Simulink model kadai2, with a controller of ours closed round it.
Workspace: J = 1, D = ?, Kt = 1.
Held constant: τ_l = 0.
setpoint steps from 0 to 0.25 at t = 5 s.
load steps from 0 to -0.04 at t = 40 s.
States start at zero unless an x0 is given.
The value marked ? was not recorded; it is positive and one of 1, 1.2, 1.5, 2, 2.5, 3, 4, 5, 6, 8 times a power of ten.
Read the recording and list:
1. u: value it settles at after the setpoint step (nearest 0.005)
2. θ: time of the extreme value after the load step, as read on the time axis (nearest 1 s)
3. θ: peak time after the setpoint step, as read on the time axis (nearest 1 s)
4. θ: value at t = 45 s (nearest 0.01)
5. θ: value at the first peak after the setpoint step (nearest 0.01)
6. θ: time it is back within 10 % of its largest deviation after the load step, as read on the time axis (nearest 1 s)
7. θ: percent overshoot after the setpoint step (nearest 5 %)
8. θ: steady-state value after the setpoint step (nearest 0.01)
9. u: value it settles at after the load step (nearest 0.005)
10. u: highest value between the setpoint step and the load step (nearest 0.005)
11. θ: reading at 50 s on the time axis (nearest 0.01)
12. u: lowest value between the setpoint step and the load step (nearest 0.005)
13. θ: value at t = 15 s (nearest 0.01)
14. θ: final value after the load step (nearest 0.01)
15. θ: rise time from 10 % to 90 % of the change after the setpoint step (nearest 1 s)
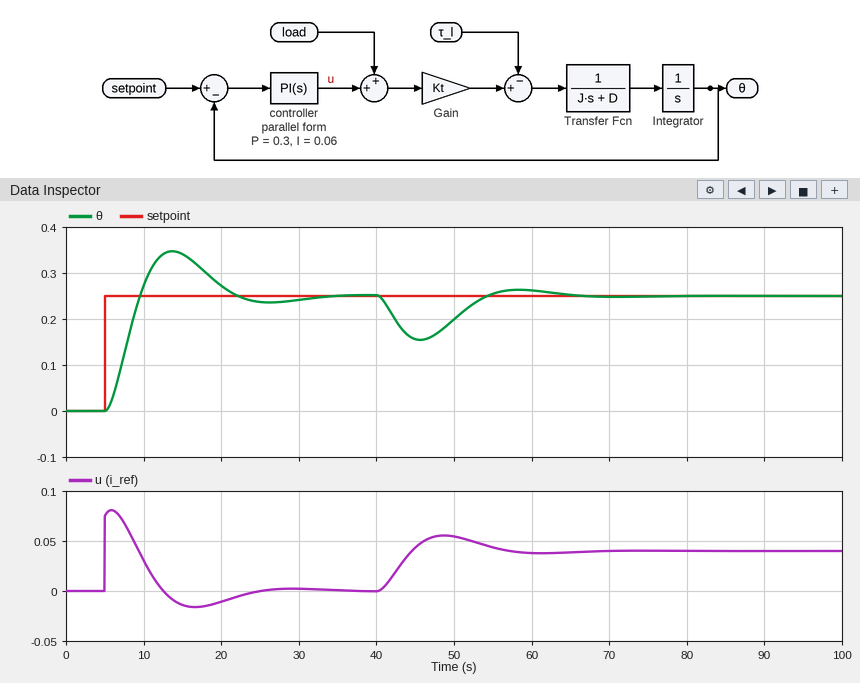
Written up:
0.000
46 s
14 s
0.16
0.35
61 s
40 %
0.25
0.040
0.080
0.20
-0.015
0.34
0.25
3 s
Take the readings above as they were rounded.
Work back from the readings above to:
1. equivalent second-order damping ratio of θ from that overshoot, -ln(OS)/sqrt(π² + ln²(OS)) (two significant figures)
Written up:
0.28
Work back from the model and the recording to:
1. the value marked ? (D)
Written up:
1
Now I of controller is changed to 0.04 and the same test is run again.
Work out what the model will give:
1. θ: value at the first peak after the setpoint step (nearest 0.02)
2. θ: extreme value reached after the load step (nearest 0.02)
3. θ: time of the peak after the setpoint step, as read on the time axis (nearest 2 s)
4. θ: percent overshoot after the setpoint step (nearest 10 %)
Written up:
0.32
0.14
14 s
30 %
